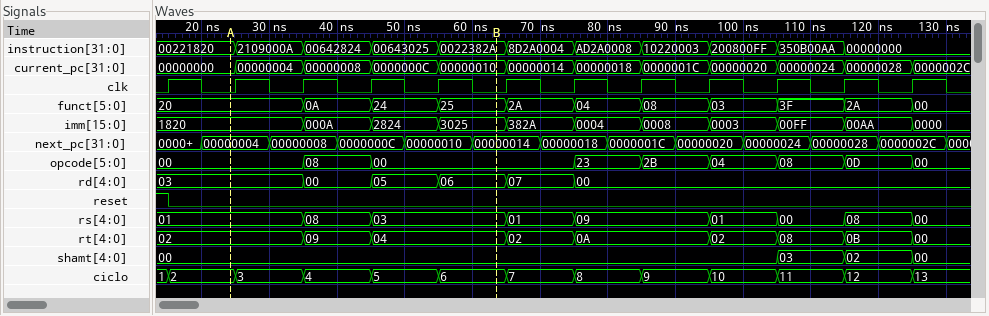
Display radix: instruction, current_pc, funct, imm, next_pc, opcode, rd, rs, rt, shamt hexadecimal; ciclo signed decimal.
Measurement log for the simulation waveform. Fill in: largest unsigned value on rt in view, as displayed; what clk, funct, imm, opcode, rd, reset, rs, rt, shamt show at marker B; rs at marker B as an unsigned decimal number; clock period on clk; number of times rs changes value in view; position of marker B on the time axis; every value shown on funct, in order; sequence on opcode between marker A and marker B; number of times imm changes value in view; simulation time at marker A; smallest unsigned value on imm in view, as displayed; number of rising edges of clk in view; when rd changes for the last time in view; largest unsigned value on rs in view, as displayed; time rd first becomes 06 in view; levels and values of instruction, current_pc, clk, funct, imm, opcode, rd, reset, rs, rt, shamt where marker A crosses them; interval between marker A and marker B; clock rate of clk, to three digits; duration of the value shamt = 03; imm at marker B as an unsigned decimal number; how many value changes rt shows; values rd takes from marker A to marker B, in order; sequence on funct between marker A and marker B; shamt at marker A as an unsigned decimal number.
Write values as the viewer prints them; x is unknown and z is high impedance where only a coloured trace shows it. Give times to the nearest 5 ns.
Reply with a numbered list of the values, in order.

1. 0B
2. clk=0, funct=25, imm=3025, opcode=00, rd=06, reset=0, rs=03, rt=04, shamt=00
3. 3
4. 10 ns
5. 8
6. 65 ns
7. 20, 0A, 24, 25, 2A, 04, 08, 03, 3F, 2A, 00
8. 00, 08, 00
9. 10
10. 25 ns
11. 0000
12. 12
13. 75 ns
14. 09
15. 55 ns
16. instruction=00221820, current_pc=00000000, clk=0, funct=20, imm=1820, opcode=00, rd=03, reset=0, rs=01, rt=02, shamt=00
17. 40 ns
18. 100 MHz
19. 10 ns
20. 12325
21. 8
22. 03, 00, 05, 06
23. 20, 0A, 24, 25
24. 0
